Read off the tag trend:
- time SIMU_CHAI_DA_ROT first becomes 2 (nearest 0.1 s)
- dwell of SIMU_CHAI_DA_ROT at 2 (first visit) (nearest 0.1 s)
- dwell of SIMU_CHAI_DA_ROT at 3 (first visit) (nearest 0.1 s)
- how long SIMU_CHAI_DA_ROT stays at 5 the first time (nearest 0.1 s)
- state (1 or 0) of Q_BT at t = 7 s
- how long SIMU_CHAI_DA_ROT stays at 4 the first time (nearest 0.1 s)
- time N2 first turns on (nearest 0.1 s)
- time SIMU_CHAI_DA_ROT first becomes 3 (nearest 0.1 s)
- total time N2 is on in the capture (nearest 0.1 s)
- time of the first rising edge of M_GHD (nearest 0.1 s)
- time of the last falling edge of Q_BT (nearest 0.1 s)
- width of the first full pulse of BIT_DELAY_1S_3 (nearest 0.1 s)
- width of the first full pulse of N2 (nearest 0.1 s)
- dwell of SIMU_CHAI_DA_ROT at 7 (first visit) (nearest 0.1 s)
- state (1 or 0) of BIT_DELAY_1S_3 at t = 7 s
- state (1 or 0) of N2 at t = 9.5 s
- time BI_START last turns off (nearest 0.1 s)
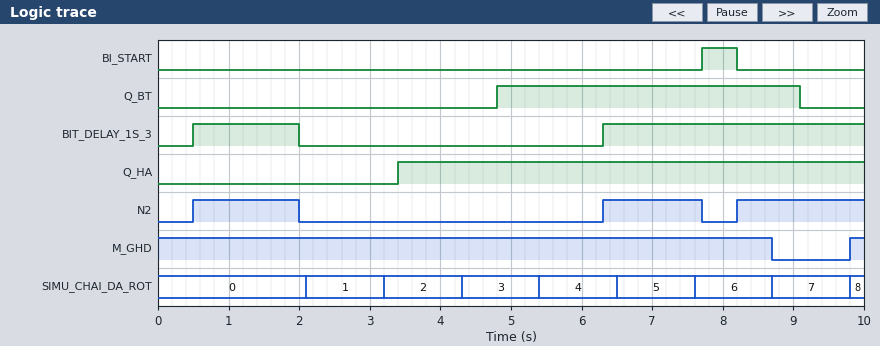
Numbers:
3.2 s
1.1 s
1.1 s
1.1 s
1
1.1 s
0.5 s
4.3 s
4.7 s
9.8 s
9.1 s
1.5 s
1.5 s
1.1 s
1
1
8.2 s
